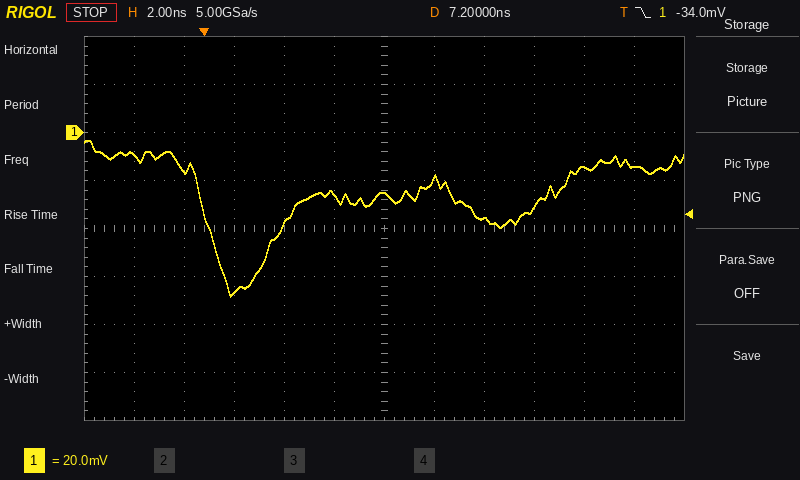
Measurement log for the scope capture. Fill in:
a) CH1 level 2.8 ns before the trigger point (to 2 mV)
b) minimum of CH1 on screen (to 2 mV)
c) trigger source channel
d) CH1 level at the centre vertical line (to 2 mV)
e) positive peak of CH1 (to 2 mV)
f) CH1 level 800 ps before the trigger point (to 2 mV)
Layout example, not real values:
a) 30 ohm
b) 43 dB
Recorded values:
a) -10 mV
b) -68 mV
c) CH1
d) -26 mV
e) -4 mV
f) -16 mV
